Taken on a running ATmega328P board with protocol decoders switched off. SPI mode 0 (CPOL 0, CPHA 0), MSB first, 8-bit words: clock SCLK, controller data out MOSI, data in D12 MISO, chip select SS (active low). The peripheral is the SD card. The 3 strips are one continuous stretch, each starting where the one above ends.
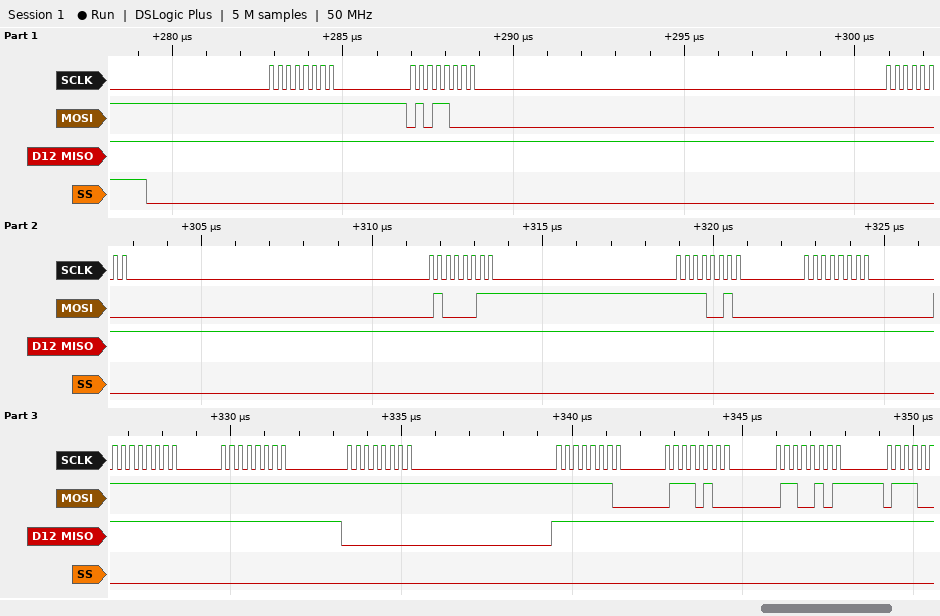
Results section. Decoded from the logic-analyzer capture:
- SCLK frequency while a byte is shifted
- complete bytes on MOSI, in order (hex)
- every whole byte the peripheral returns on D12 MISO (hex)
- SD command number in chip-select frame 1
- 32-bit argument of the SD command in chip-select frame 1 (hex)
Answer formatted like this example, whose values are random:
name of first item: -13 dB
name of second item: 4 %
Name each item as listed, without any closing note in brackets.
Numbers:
SCLK frequency while a byte is shifted: 4 MHz
complete bytes on MOSI, in order: 0xFF 0x58 0x00 0x43 0xF2 0x00 0xFF 0xFF 0xFF 0xFE 0x74 0x65
every whole byte the peripheral returns on D12 MISO: 0xFF 0xFF 0xFF 0xFF 0xFF 0xFF 0xFF 0xFF 0x00 0xFF 0xFF 0xFF
SD command number in chip-select frame 1: CMD24
32-bit argument of the SD command in chip-select frame 1: 0x0043F200
